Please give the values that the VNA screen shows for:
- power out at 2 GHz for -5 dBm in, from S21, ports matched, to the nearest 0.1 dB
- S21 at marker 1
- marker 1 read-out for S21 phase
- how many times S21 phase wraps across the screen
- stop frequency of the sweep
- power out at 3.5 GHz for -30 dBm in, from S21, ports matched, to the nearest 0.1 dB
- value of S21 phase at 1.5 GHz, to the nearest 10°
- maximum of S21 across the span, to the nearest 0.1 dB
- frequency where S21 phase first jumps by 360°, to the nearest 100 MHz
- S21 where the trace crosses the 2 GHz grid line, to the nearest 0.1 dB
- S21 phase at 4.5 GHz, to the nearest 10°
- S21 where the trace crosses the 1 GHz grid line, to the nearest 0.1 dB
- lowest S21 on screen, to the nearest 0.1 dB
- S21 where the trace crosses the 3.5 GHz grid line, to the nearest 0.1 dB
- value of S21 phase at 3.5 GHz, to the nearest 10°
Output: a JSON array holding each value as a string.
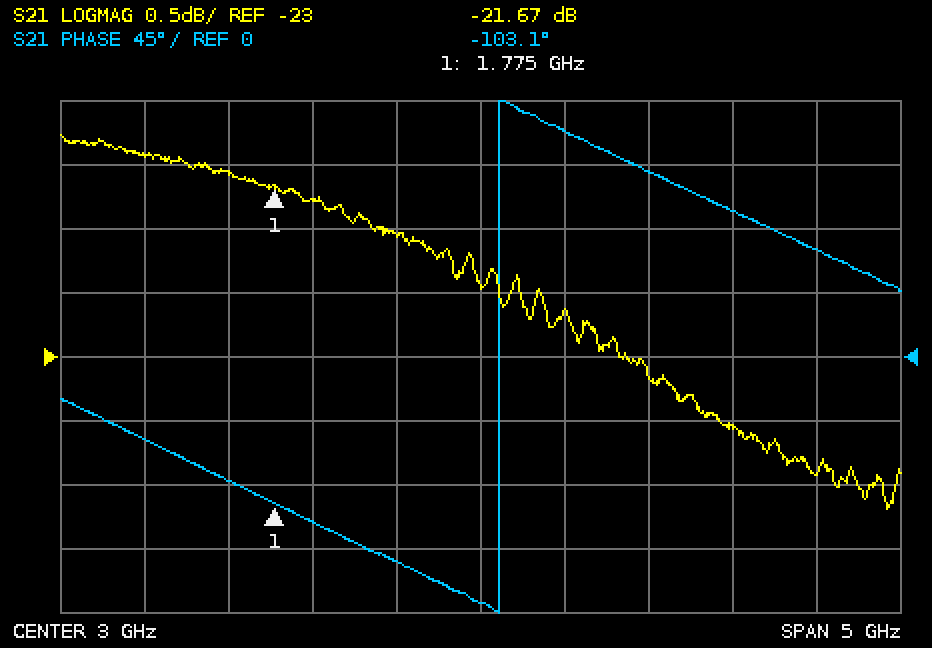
["-26.8 dBm", "-21.67 dB", "-103.1°", "1", "5.5 GHz", "-52.6 dBm", "-90°", "-21.3 dB", "3.1 GHz", "-21.8 dB", "100°", "-21.4 dB", "-24.2 dB", "-22.6 dB", "160°"]
